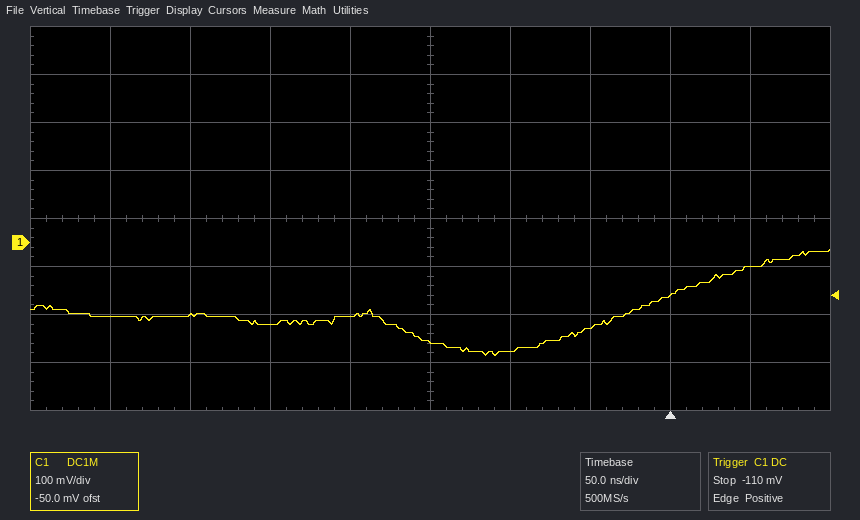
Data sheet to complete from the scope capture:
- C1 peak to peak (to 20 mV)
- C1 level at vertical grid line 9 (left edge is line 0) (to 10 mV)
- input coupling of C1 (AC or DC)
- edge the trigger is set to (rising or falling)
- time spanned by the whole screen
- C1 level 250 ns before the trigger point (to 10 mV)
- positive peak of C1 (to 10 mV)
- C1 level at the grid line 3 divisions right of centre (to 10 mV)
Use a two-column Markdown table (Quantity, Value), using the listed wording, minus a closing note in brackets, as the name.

| Quantity | Value |
|---|---|
| C1 peak to peak | 220 mV |
| C1 level at vertical grid line 9 (left edge is line 0) | -50 mV |
| input coupling of C1 | DC |
| edge the trigger is set to | rising |
| time spanned by the whole screen | 500 ns |
| C1 level 250 ns before the trigger point | -170 mV |
| positive peak of C1 | -10 mV |
| C1 level at the grid line 3 divisions right of centre | -110 mV |
